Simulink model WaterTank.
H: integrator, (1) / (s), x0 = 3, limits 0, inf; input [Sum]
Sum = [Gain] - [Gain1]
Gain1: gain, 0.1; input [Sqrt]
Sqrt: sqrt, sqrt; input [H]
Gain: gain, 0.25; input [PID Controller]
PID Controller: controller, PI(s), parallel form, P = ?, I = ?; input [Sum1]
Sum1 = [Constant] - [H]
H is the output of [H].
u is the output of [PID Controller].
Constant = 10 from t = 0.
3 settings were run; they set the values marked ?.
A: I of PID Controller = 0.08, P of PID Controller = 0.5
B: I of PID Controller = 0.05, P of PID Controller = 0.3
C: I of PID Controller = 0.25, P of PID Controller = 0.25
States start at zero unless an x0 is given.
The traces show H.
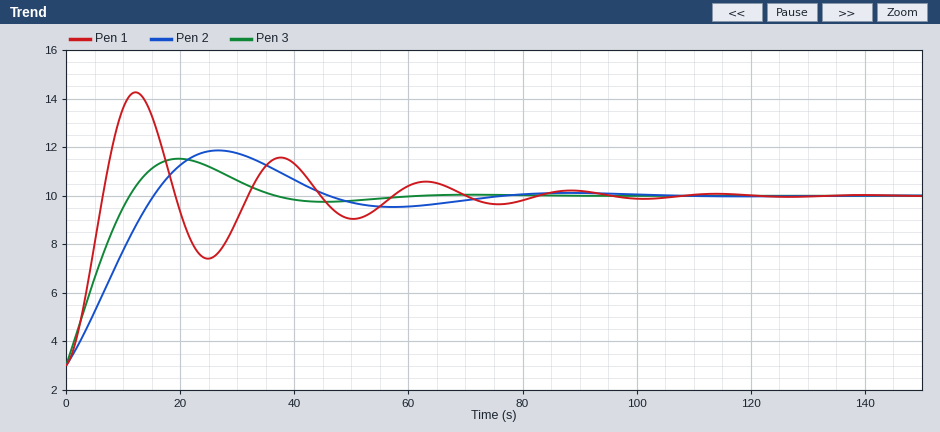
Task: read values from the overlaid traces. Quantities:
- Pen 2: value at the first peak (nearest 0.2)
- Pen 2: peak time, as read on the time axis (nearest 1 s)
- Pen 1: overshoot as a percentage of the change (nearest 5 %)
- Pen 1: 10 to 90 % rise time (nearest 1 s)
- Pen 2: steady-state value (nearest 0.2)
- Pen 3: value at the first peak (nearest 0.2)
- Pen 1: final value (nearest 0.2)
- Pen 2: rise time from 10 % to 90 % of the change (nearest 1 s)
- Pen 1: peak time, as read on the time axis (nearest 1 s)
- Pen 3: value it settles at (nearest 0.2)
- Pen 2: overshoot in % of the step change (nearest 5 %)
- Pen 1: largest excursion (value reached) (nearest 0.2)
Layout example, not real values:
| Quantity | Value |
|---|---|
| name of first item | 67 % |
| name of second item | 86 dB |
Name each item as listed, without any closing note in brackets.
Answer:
| Quantity | Value |
|---|---|
| Pen 2: value at the first peak | 11.8 |
| Pen 2: peak time, as read on the time axis | 27 s |
| Pen 1: overshoot as a percentage of the change | 60 % |
| Pen 1: 10 to 90 % rise time | 5 s |
| Pen 2: steady-state value | 10.0 |
| Pen 3: value at the first peak | 11.6 |
| Pen 1: final value | 10.0 |
| Pen 2: rise time from 10 % to 90 % of the change | 12 s |
| Pen 1: peak time, as read on the time axis | 12 s |
| Pen 3: value it settles at | 10.0 |
| Pen 2: overshoot in % of the step change | 25 % |
| Pen 1: largest excursion (value reached) | 14.2 |
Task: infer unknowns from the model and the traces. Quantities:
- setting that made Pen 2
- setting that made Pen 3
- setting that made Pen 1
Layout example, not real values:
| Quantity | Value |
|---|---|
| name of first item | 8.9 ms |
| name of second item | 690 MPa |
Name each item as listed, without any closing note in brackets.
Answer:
| Quantity | Value |
|---|---|
| setting that made Pen 2 | B |
| setting that made Pen 3 | A |
| setting that made Pen 1 | C |
